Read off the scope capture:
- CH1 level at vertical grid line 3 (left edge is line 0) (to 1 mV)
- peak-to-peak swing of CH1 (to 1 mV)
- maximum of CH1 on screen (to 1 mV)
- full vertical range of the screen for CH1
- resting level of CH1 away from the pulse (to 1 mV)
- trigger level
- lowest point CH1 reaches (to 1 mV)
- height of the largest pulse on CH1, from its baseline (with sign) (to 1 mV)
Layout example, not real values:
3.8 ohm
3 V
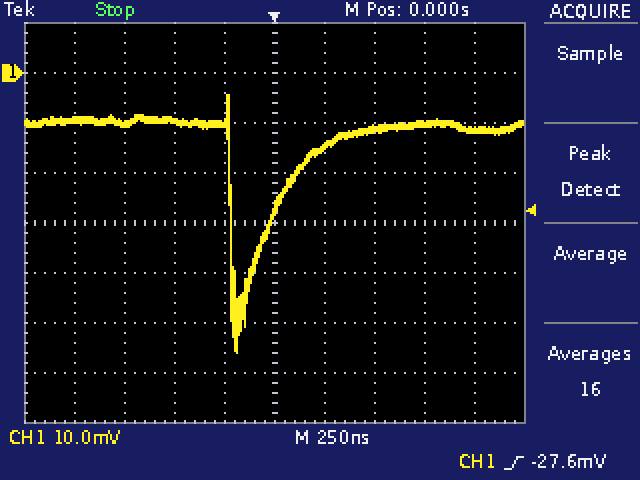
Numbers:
-10 mV
52 mV
-4 mV
80 mV
-10 mV
-27.6 mV
-56 mV
-46 mV
